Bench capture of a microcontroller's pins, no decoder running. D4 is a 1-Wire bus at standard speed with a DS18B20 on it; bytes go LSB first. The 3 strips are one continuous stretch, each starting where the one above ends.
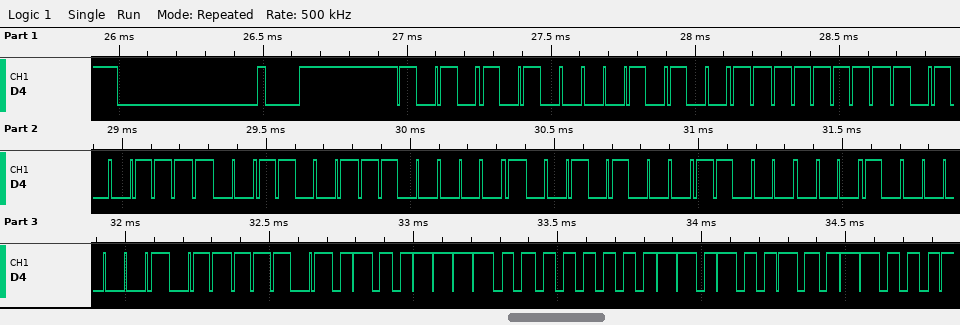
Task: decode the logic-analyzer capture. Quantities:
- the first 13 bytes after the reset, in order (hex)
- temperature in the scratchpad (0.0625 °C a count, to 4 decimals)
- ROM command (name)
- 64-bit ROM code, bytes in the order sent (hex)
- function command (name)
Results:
55 28 FF E5 99 83 14 03 81 BE F2 00 4B
15.1250 °C
Match ROM
28 FF E5 99 83 14 03 81
Read Scratchpad
